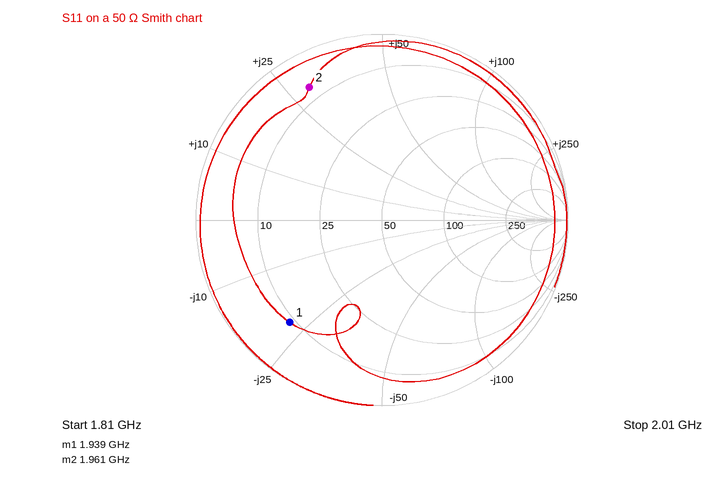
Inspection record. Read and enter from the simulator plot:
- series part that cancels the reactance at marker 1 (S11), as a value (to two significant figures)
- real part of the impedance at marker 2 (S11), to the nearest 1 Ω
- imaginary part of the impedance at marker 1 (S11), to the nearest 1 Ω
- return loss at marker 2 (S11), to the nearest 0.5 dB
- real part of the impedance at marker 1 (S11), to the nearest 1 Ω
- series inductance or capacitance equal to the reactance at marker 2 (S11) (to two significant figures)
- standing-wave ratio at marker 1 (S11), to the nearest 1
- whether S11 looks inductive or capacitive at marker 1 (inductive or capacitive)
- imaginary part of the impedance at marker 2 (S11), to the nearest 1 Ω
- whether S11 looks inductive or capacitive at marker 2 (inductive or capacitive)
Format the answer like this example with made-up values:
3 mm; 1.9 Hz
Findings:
1.8 nH; 7 Ω; -22 Ω; 2.0 dB; 9 Ω; 2.4 nH; 7; capacitive; +29 Ω; inductive
